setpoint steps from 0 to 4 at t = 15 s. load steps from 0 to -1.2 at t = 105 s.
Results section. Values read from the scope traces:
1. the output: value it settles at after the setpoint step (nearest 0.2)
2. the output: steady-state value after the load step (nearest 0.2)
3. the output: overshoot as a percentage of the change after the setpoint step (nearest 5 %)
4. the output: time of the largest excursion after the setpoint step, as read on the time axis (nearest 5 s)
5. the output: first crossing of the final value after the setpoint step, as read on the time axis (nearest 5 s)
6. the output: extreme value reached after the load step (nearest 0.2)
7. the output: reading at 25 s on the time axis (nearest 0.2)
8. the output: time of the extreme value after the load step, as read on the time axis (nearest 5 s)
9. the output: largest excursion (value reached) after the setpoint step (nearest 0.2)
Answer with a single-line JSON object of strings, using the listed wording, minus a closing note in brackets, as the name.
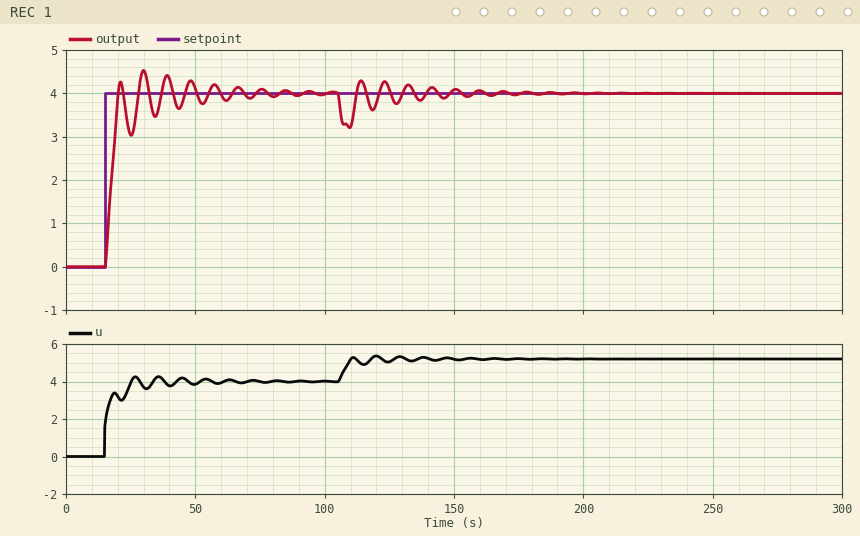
{"the output: value it settles at after the setpoint step": "4.0", "the output: steady-state value after the load step": "4.0", "the output: overshoot as a percentage of the change after the setpoint step": "15 %", "the output: time of the largest excursion after the setpoint step, as read on the time axis": "30 s", "the output: first crossing of the final value after the setpoint step, as read on the time axis": "20 s", "the output: extreme value reached after the load step": "3.2", "the output: reading at 25 s on the time axis": "3.0", "the output: time of the extreme value after the load step, as read on the time axis": "110 s", "the output: largest excursion (value reached) after the setpoint step": "4.6"}
